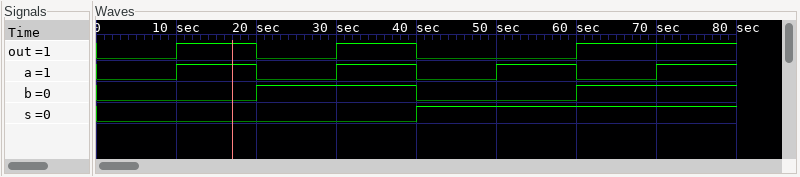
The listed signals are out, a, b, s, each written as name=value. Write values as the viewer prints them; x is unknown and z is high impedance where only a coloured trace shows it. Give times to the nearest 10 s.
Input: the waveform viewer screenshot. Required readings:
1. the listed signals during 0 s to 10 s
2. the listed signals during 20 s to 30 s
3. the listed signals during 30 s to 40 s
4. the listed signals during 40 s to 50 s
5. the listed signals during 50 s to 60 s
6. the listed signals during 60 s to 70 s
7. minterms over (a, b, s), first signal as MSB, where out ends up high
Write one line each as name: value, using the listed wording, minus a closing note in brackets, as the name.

the listed signals during 0 s to 10 s: out=0, a=0, b=0, s=0
the listed signals during 20 s to 30 s: out=0, a=0, b=1, s=0
the listed signals during 30 s to 40 s: out=1, a=1, b=1, s=0
the listed signals during 40 s to 50 s: out=0, a=0, b=0, s=1
the listed signals during 50 s to 60 s: out=0, a=1, b=0, s=1
the listed signals during 60 s to 70 s: out=1, a=0, b=1, s=1
minterms over (a, b, s), first signal as MSB, where out ends up high: 3, 4, 6, 7
